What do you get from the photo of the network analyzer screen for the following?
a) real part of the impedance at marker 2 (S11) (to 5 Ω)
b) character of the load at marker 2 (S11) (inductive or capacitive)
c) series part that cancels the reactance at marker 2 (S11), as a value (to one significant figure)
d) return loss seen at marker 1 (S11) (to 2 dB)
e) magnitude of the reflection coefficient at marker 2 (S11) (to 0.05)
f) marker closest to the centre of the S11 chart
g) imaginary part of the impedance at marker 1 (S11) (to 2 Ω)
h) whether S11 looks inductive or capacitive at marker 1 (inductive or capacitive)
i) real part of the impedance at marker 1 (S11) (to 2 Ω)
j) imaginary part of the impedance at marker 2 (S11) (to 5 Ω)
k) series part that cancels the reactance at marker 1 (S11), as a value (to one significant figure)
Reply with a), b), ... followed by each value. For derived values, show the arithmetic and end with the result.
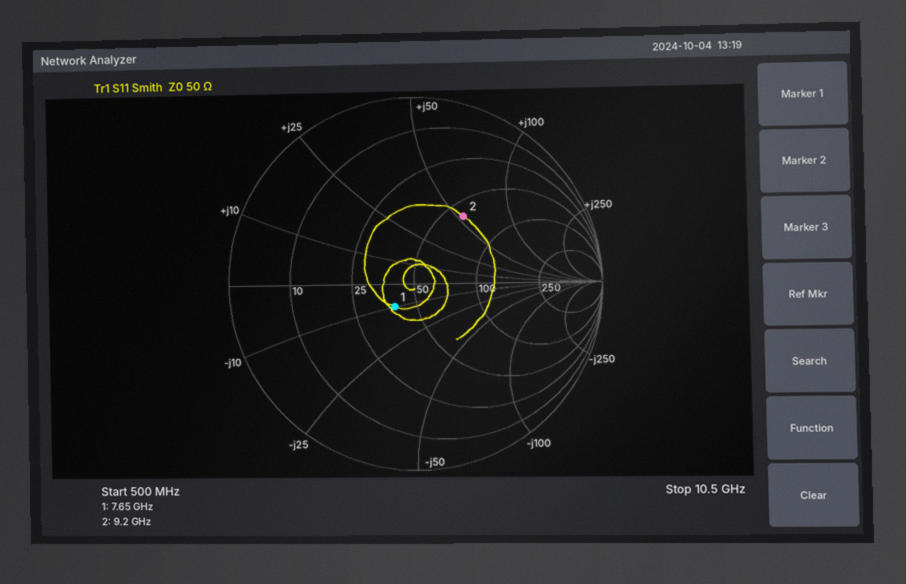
a) 60 Ω
b) inductive
c) C = 1/(2π × 9.2 GHz × 55 Ω) ≈ 315 fF, so 300 fF to one significant figure
d) 16 dB
e) 0.45
f) marker 1
g) -10 Ω
h) capacitive
i) 40 Ω
j) +55 Ω
k) L = 10 Ω/(2π × 7.65 GHz) ≈ 208 pH, so 200 pH to one significant figure
